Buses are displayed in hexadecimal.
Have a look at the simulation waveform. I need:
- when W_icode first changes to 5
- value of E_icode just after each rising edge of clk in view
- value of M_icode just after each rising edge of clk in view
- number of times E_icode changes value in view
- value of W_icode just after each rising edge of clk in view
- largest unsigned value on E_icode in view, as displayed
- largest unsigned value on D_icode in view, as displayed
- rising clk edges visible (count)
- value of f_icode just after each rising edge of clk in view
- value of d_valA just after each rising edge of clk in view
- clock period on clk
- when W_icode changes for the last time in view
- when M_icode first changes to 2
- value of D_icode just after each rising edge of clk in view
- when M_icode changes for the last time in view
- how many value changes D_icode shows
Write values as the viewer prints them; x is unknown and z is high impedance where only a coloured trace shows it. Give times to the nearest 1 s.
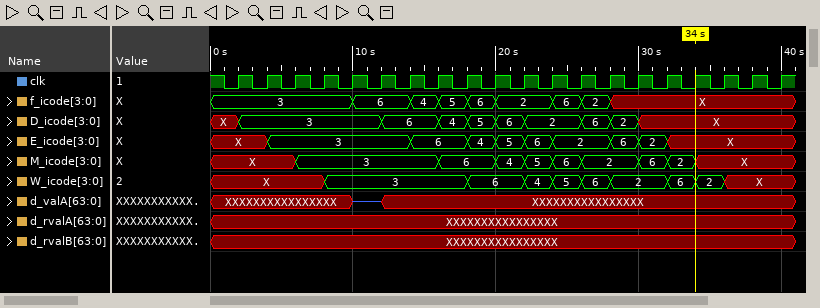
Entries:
24 s
X, 3, 3, 3, 3, 3, 6, 6, 4, 5, 6, 2, 2, 6, 2, X, X, X, X, X
X, X, 3, 3, 3, 3, 3, 6, 6, 4, 5, 6, 2, 2, 6, 2, X, X, X, X
9
X, X, X, 3, 3, 3, 3, 3, 6, 6, 4, 5, 6, 2, 2, 6, 2, X, X, X
6
6
20
3, 3, 3, 3, 6, 6, 4, 5, 6, 2, 2, 6, 2, X, X, X, X, X, X, X
XXXXXXXXXXXXXXXX, XXXXXXXXXXXXXXXX, XXXXXXXXXXXXXXXX, XXXXXXXXXXXXXXXX, z, XXXXXXXXXXXXXXXX, XXXXXXXXXXXXXXXX, XXXXXXXXXXXXXXXX, XXXXXXXXXXXXXXXX, XXXXXXXXXXXXXXXX, XXXXXXXXXXXXXXXX, XXXXXXXXXXXXXXXX, XXXXXXXXXXXXXXXX, XXXXXXXXXXXXXXXX, XXXXXXXXXXXXXXXX, XXXXXXXXXXXXXXXX, XXXXXXXXXXXXXXXX, XXXXXXXXXXXXXXXX, XXXXXXXXXXXXXXXX, XXXXXXXXXXXXXXXX
2 s
36 s
26 s
3, 3, 3, 3, 3, 6, 6, 4, 5, 6, 2, 2, 6, 2, X, X, X, X, X, X
34 s
9
